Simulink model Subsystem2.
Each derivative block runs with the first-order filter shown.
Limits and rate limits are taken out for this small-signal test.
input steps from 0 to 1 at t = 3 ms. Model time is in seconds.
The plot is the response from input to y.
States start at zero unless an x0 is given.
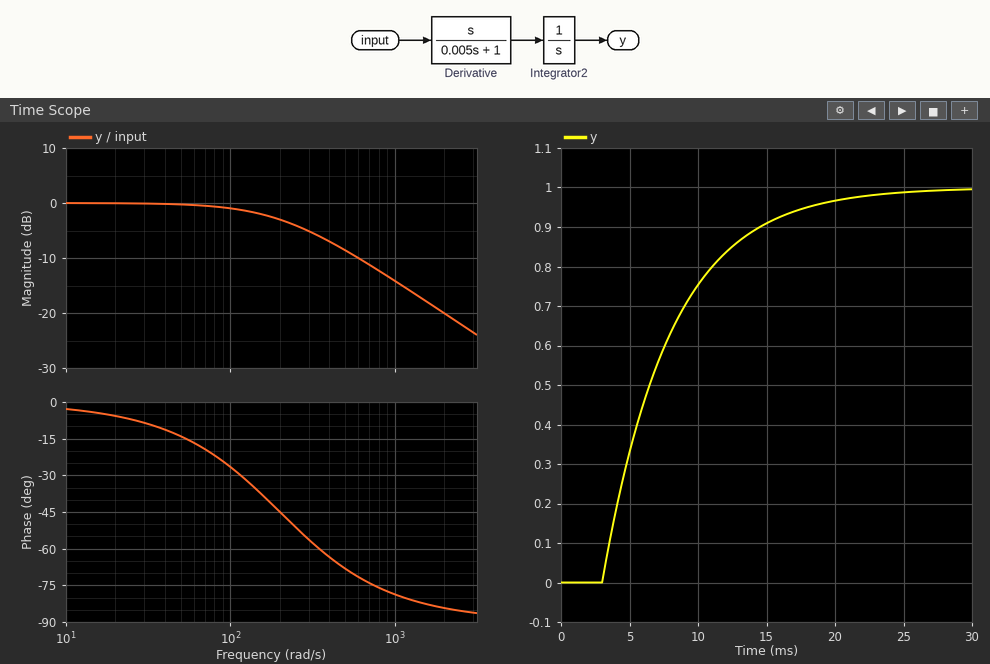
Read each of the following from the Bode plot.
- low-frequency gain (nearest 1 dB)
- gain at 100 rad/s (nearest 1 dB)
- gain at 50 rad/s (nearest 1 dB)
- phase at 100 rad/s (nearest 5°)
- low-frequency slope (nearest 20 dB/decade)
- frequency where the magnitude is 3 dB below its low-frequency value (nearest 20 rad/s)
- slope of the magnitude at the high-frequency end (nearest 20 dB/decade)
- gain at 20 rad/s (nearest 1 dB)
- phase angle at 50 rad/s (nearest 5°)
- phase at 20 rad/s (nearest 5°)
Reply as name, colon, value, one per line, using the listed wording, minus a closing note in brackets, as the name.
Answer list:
low-frequency gain: 0 dB
gain at 100 rad/s: -1 dB
gain at 50 rad/s: 0 dB
phase at 100 rad/s: -25°
low-frequency slope: 0 dB/decade
frequency where the magnitude is 3 dB below its low-frequency value: 200 rad/s
slope of the magnitude at the high-frequency end: -20 dB/decade
gain at 20 rad/s: 0 dB
phase angle at 50 rad/s: -15°
phase at 20 rad/s: -5°
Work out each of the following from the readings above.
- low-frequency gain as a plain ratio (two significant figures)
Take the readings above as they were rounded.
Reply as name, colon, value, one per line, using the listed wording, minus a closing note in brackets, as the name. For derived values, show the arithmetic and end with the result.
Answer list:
low-frequency gain as a plain ratio: 10^(0 / 20) = 1.0
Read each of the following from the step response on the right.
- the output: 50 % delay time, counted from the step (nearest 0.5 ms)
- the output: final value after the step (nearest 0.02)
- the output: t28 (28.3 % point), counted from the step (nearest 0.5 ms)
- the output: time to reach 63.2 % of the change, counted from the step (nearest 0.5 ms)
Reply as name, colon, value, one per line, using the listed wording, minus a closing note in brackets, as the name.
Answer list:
the output: 50 % delay time, counted from the step: 3.5 ms
the output: final value after the step: 1.00
the output: t28 (28.3 % point), counted from the step: 1.5 ms
the output: time to reach 63.2 % of the change, counted from the step: 5.0 ms
